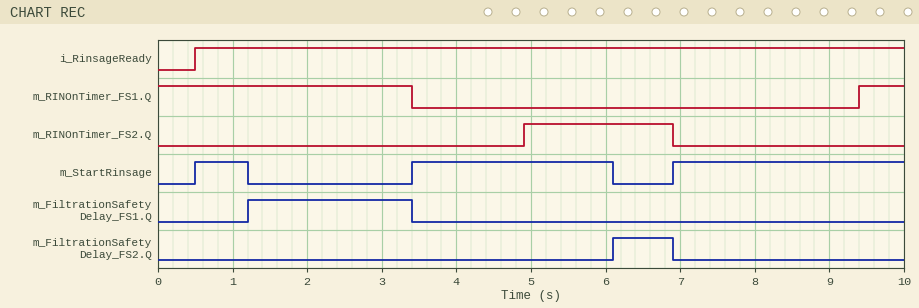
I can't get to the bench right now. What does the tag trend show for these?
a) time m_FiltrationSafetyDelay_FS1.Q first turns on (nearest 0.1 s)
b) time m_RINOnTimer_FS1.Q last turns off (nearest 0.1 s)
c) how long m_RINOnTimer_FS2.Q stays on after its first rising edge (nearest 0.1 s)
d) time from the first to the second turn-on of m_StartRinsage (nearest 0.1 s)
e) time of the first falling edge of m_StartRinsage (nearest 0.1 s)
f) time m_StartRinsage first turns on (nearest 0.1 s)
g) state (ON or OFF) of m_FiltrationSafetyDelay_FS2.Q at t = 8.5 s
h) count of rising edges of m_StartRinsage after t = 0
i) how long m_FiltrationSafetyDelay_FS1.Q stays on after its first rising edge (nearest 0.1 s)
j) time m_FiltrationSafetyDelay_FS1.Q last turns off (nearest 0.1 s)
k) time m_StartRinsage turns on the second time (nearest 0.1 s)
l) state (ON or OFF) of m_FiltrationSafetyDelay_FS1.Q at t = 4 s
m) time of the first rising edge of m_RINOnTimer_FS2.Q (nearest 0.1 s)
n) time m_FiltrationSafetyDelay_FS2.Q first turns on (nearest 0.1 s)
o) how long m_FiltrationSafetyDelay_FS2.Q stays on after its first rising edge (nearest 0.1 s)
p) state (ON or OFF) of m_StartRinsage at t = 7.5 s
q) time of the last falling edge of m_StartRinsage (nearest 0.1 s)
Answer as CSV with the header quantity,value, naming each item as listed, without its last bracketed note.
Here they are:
quantity,value
time m_FiltrationSafetyDelay_FS1.Q first turns on,1.2 s
time m_RINOnTimer_FS1.Q last turns off,3.4 s
how long m_RINOnTimer_FS2.Q stays on after its first rising edge,2.0 s
time from the first to the second turn-on of m_StartRinsage,2.9 s
time of the first falling edge of m_StartRinsage,1.2 s
time m_StartRinsage first turns on,0.5 s
state (ON or OFF) of m_FiltrationSafetyDelay_FS2.Q at t = 8.5 s,OFF
count of rising edges of m_StartRinsage after t = 0,3
how long m_FiltrationSafetyDelay_FS1.Q stays on after its first rising edge,2.2 s
time m_FiltrationSafetyDelay_FS1.Q last turns off,3.4 s
time m_StartRinsage turns on the second time,3.4 s
state (ON or OFF) of m_FiltrationSafetyDelay_FS1.Q at t = 4 s,OFF
time of the first rising edge of m_RINOnTimer_FS2.Q,4.9 s
time m_FiltrationSafetyDelay_FS2.Q first turns on,6.1 s
how long m_FiltrationSafetyDelay_FS2.Q stays on after its first rising edge,0.8 s
state (ON or OFF) of m_StartRinsage at t = 7.5 s,ON
time of the last falling edge of m_StartRinsage,6.1 s
